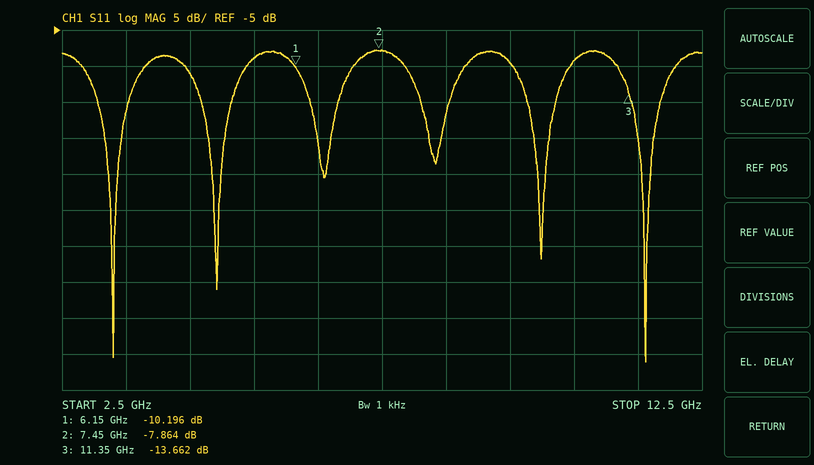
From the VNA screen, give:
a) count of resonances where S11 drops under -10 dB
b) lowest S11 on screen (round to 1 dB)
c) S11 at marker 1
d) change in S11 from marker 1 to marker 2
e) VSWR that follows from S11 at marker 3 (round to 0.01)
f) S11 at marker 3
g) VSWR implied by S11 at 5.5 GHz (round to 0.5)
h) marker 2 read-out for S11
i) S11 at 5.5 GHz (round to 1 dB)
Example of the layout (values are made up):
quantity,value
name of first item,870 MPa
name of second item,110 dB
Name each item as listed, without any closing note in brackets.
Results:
quantity,value
count of resonances where S11 drops under -10 dB,6
lowest S11 on screen,-51 dB
S11 at marker 1,-10.196 dB
change in S11 from marker 1 to marker 2,2.332 dB
VSWR that follows from S11 at marker 3,1.52
S11 at marker 3,-13.662 dB
VSWR implied by S11 at 5.5 GHz,2.0
marker 2 read-out for S11,-7.864 dB
S11 at 5.5 GHz,-9 dB
